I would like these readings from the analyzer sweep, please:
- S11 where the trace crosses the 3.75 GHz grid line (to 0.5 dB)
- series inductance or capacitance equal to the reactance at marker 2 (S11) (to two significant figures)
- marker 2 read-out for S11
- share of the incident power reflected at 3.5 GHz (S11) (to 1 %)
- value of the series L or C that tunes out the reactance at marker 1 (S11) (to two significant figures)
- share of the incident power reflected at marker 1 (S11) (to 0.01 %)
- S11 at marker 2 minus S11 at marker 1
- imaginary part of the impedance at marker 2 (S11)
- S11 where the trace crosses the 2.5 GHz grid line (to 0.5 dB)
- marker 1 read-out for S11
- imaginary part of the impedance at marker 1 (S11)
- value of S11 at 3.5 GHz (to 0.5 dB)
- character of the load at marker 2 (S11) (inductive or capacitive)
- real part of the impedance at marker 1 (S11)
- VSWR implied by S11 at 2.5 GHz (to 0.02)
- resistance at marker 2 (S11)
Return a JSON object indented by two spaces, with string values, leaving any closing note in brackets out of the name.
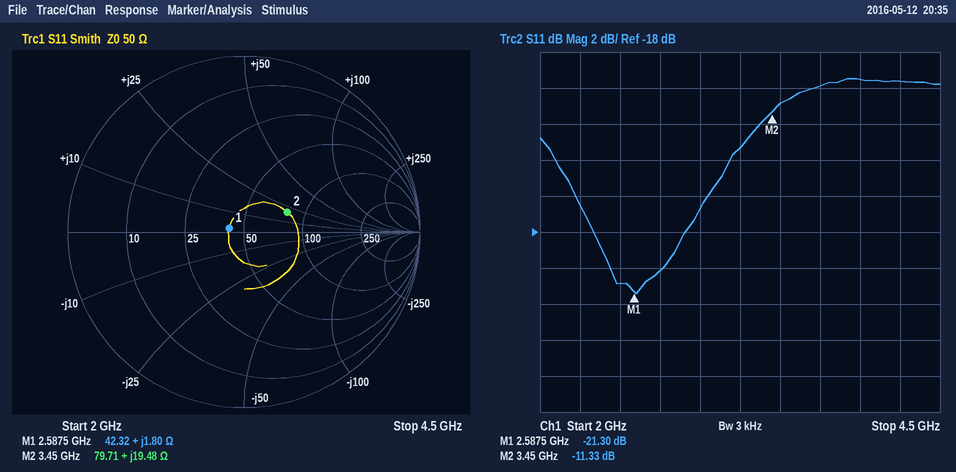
{
  "S11 where the trace crosses the 3.75 GHz grid line": "-10.0 dB",
  "series inductance or capacitance equal to the reactance at marker 2 (S11)": "900 pH",
  "marker 2 read-out for S11": "-11.33 dB",
  "share of the incident power reflected at 3.5 GHz (S11)": "8 %",
  "value of the series L or C that tunes out the reactance at marker 1 (S11)": "34 pF",
  "share of the incident power reflected at marker 1 (S11)": "0.74 %",
  "S11 at marker 2 minus S11 at marker 1": "9.97 dB",
  "imaginary part of the impedance at marker 2": "+19.48 Ω",
  "S11 where the trace crosses the 2.5 GHz grid line": "-21.0 dB",
  "marker 1 read-out for S11": "-21.30 dB",
  "imaginary part of the impedance at marker 1": "+1.80 Ω",
  "value of S11 at 3.5 GHz": "-11.0 dB",
  "character of the load at marker 2 (S11)": "inductive",
  "real part of the impedance at marker 1": "42.32 Ω",
  "VSWR implied by S11 at 2.5 GHz": "1.20",
  "resistance at marker 2": "79.71 Ω"
}
